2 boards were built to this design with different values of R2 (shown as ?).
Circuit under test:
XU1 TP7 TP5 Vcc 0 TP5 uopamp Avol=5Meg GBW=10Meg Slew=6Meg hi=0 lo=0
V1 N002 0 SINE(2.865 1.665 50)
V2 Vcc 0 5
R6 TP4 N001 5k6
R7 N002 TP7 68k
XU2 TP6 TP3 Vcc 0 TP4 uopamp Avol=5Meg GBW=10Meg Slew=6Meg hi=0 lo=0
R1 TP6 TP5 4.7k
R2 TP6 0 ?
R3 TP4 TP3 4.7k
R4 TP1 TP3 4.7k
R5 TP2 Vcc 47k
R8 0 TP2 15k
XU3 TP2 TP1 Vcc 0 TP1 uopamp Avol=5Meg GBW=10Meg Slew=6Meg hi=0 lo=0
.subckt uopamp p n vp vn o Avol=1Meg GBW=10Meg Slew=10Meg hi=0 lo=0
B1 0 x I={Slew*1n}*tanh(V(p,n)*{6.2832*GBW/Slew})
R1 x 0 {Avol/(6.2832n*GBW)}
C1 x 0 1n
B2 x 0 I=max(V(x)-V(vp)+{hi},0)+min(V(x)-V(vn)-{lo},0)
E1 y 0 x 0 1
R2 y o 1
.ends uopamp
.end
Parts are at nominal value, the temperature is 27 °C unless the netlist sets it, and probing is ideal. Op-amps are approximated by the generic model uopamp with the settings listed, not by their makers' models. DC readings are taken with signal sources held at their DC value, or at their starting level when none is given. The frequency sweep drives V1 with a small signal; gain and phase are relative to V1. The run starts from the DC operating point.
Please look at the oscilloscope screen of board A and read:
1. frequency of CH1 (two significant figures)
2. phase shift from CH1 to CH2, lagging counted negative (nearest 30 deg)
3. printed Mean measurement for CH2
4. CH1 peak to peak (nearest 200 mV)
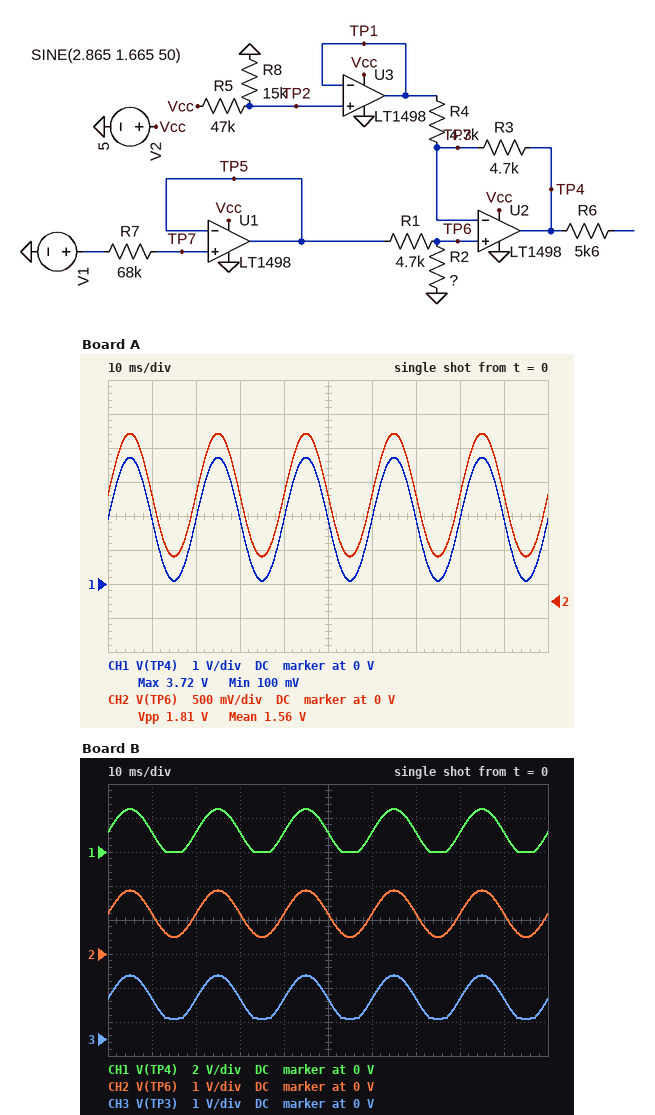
50 Hz
0 deg
1.56 V
3.6 V
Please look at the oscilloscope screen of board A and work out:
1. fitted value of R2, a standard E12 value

5.6 kΩ
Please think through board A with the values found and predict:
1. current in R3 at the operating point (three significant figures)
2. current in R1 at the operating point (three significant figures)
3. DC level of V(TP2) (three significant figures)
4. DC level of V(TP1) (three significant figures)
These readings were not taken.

74.0 µA
278 µA
1.21 V
1.21 V
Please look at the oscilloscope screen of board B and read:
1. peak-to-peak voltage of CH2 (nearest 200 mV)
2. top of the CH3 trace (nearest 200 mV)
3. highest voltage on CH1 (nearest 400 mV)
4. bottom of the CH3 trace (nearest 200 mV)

1.4 V
1.8 V
2.4 V
600 mV
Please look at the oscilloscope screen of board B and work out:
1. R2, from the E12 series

3.3 kΩ
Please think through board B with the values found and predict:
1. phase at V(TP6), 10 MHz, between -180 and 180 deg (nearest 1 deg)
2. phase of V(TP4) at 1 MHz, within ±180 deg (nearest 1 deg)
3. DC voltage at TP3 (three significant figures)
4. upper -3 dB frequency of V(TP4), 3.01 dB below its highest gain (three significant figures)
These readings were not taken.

-45 deg
-17 deg
1.18 V
4.19 MHz
